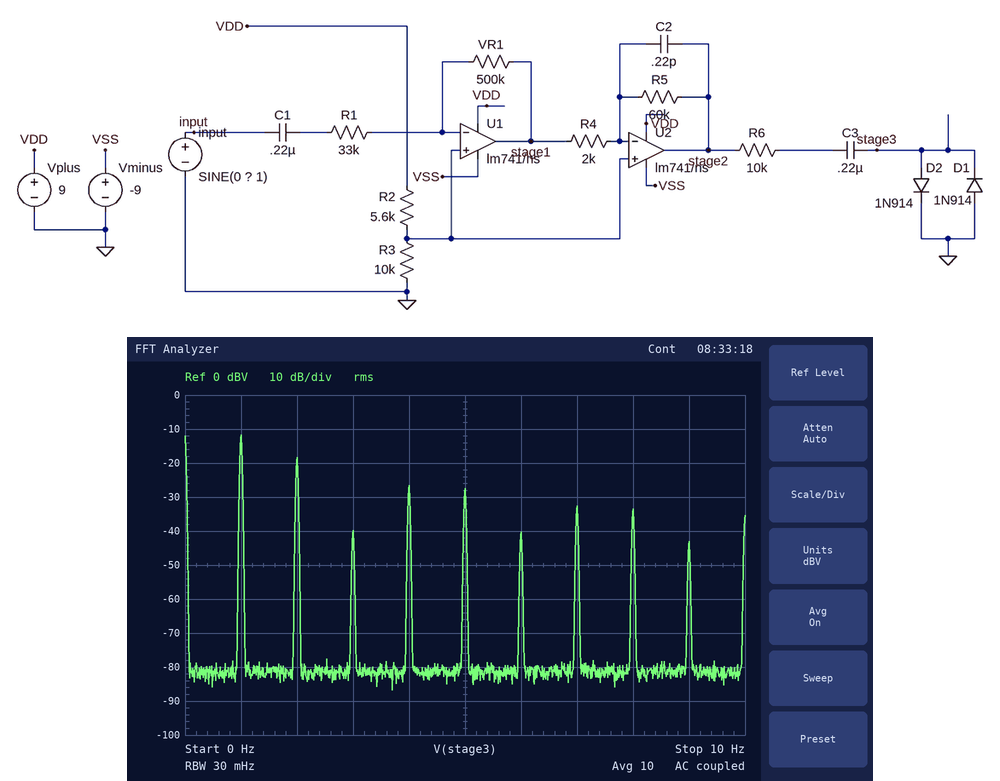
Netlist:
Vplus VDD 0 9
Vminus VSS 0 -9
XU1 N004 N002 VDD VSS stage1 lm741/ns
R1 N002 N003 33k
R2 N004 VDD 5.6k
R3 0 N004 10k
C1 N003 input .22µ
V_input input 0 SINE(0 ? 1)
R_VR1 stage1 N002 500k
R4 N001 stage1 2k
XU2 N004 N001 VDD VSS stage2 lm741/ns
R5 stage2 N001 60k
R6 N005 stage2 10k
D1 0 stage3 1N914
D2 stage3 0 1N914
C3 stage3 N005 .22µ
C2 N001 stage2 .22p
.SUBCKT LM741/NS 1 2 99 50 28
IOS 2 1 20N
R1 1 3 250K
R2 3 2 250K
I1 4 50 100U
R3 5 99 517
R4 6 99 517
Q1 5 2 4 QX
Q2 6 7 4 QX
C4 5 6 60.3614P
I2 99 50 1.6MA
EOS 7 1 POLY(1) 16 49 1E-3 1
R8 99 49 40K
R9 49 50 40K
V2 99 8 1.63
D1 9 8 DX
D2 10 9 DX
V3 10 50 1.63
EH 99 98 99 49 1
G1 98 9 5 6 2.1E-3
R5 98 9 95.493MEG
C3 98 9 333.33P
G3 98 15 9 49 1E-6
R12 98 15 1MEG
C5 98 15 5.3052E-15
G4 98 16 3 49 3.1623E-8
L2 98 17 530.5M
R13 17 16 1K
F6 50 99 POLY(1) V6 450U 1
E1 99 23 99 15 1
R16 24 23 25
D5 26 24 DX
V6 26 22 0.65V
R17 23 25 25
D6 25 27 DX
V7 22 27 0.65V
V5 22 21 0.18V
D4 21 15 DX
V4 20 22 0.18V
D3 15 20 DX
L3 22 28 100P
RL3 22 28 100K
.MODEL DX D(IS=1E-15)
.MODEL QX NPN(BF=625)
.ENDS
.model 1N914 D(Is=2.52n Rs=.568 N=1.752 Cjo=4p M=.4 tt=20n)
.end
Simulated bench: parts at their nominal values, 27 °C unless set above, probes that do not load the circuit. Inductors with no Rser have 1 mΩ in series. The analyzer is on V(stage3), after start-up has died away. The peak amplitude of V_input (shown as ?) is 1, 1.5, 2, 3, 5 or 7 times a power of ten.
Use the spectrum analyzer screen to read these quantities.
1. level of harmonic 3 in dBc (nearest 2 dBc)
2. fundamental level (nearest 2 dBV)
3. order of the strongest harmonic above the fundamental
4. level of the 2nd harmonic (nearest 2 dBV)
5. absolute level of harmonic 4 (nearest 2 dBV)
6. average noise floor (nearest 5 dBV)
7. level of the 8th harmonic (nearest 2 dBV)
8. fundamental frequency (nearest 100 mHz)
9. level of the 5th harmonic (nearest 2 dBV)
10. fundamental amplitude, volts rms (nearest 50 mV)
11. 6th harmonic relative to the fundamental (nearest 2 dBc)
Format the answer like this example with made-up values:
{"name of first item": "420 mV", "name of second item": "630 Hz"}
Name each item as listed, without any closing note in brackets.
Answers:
{"level of harmonic 3 in dBc": "-28 dBc", "fundamental level": "-12 dBV", "order of the strongest harmonic above the fundamental": "2", "level of the 2nd harmonic": "-18 dBV", "absolute level of harmonic 4": "-26 dBV", "average noise floor": "-80 dBV", "level of the 8th harmonic": "-34 dBV", "fundamental frequency": "1.0 Hz", "level of the 5th harmonic": "-28 dBV", "fundamental amplitude, volts rms": "250 mV", "6th harmonic relative to the fundamental": "-28 dBc"}
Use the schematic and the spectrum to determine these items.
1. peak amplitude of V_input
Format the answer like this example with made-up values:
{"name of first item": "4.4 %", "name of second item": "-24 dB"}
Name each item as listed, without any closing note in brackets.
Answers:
{"peak amplitude of V_input": "500 mV"}
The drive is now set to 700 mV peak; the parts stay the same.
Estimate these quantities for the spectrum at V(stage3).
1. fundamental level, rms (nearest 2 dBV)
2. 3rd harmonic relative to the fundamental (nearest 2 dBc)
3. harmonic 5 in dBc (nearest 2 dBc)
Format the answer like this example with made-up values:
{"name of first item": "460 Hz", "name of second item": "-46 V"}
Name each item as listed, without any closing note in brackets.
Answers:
{"fundamental level, rms": "-12 dBV", "3rd harmonic relative to the fundamental": "-14 dBc", "harmonic 5 in dBc": "-28 dBc"}
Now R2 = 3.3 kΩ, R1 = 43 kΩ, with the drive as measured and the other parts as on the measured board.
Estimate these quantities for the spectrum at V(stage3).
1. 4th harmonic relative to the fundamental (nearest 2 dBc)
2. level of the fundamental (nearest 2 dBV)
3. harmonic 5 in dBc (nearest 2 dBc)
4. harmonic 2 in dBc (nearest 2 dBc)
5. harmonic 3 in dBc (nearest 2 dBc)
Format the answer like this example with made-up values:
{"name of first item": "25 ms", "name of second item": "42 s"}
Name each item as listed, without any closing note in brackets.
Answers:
{"4th harmonic relative to the fundamental": "-16 dBc", "level of the fundamental": "-12 dBV", "harmonic 5 in dBc": "-14 dBc", "harmonic 2 in dBc": "-6 dBc", "harmonic 3 in dBc": "-42 dBc"}
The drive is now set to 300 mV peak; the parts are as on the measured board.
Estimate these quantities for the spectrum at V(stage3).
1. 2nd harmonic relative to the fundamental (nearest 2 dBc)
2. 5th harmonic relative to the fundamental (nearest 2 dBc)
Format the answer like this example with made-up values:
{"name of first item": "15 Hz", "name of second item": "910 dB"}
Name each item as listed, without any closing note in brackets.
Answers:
{"2nd harmonic relative to the fundamental": "-12 dBc", "5th harmonic relative to the fundamental": "-36 dBc"}
